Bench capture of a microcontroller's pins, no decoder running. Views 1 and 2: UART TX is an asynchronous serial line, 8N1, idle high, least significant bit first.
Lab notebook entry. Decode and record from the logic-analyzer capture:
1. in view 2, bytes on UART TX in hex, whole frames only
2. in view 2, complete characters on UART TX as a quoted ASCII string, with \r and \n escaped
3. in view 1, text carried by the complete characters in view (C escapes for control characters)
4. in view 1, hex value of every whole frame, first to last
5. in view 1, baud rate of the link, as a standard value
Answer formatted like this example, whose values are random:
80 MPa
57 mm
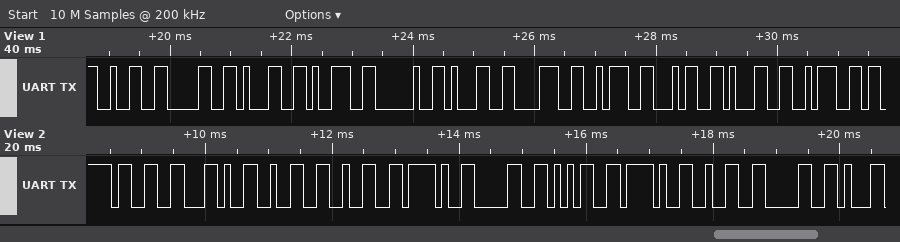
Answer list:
33 2C 32 32 2F 30 35 2F 32 30
"3,22/05/20"
"2019 18:41:"
32 30 31 39 20 31 38 3A 34 31 3A
9600 baud
